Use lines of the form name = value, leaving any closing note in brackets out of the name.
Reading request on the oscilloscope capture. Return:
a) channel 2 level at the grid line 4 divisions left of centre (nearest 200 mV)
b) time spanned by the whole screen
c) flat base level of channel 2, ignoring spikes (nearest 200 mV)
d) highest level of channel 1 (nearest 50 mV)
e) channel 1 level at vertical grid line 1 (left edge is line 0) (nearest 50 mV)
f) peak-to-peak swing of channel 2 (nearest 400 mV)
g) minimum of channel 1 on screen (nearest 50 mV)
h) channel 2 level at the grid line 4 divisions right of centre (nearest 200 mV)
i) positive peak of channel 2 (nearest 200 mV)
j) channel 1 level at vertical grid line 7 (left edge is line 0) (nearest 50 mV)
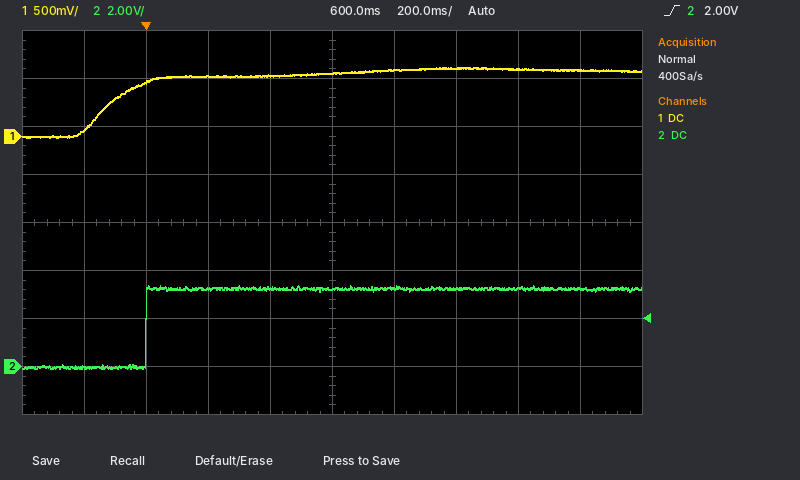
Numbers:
channel 2 level at the grid line 4 divisions left of centre = 0.0 V
time spanned by the whole screen = 2 s
flat base level of channel 2, ignoring spikes = 0.0 V
highest level of channel 1 = 700 mV
channel 1 level at vertical grid line 1 (left edge is line 0) = 50 mV
peak-to-peak swing of channel 2 = 3.6 V
minimum of channel 1 on screen = 0 mV
channel 2 level at the grid line 4 divisions right of centre = 3.2 V
positive peak of channel 2 = 3.4 V
channel 1 level at vertical grid line 7 (left edge is line 0) = 700 mV
